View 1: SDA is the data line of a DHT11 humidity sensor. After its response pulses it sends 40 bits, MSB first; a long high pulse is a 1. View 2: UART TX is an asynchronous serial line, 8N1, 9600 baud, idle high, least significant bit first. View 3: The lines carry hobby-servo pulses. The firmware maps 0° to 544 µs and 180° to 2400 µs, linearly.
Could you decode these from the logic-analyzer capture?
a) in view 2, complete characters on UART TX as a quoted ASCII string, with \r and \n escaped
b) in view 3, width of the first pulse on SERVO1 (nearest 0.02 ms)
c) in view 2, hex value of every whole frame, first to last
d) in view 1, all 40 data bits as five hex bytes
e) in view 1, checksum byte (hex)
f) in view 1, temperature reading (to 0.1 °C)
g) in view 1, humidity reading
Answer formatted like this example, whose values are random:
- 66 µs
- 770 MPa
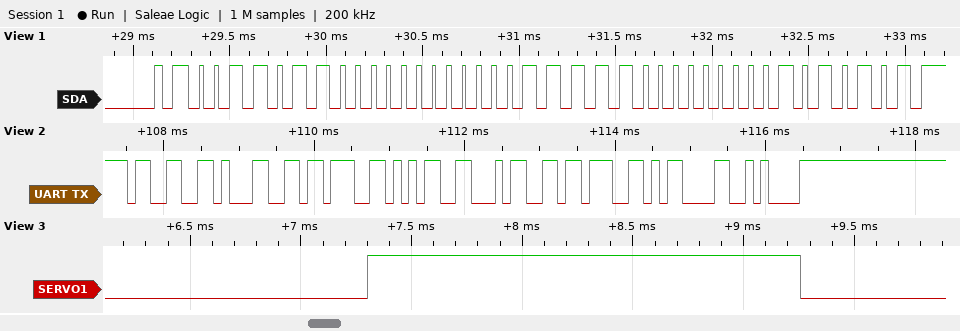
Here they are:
- "31;54;\r\n"
- 1.96 ms
- 0x33 0x31 0x3B 0x35 0x34 0x3B 0x0D 0x0A
- 36 00 1F 00 55
- 0x55
- 31.0 °C
- 54 %
